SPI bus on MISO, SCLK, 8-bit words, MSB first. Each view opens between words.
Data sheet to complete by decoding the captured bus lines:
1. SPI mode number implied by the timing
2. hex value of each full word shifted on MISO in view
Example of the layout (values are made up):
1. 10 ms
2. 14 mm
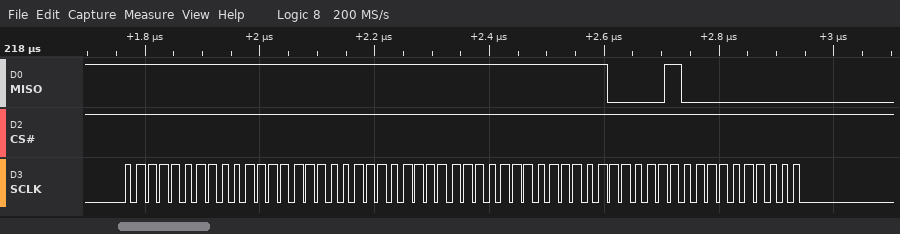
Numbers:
1. 0
2. FF, FF, FF, FF, FF, 04, 00
